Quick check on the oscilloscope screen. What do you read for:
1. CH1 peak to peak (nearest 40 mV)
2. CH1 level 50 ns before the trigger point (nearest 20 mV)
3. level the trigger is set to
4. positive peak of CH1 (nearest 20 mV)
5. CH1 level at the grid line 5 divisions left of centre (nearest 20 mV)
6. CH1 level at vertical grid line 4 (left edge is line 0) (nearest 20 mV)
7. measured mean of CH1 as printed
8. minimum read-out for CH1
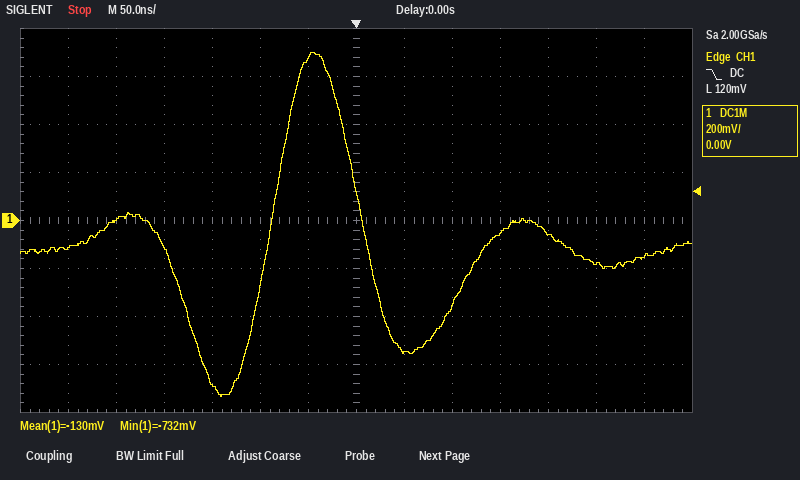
1.44 V
680 mV
120 mV
700 mV
0 mV
-680 mV
-130 mV
-732 mV
